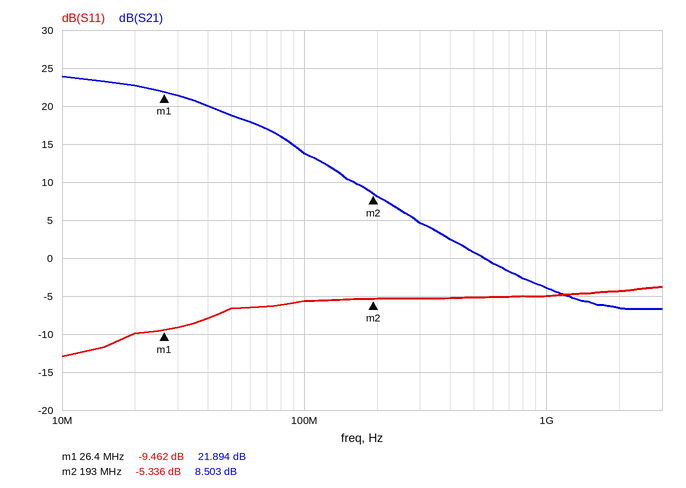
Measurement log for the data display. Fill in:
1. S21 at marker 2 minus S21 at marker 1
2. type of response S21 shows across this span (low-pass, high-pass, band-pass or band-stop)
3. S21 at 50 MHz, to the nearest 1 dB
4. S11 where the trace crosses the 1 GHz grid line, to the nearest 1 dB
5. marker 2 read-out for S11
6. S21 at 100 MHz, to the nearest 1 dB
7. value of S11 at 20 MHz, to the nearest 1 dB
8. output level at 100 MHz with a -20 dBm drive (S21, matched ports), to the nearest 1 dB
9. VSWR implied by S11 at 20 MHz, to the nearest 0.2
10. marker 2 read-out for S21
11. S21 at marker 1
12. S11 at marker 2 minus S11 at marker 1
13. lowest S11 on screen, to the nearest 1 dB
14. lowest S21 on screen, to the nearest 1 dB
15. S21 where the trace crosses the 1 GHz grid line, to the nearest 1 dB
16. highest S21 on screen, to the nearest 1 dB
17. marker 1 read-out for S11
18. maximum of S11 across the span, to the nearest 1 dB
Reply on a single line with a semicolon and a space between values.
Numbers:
-13.391 dB; low-pass; 19 dB; -5 dB; -5.336 dB; 14 dB; -10 dB; -6 dBm; 2.0; 8.503 dB; 21.894 dB; 4.126 dB; -13 dB; -7 dB; -4 dB; 24 dB; -9.462 dB; -4 dB
